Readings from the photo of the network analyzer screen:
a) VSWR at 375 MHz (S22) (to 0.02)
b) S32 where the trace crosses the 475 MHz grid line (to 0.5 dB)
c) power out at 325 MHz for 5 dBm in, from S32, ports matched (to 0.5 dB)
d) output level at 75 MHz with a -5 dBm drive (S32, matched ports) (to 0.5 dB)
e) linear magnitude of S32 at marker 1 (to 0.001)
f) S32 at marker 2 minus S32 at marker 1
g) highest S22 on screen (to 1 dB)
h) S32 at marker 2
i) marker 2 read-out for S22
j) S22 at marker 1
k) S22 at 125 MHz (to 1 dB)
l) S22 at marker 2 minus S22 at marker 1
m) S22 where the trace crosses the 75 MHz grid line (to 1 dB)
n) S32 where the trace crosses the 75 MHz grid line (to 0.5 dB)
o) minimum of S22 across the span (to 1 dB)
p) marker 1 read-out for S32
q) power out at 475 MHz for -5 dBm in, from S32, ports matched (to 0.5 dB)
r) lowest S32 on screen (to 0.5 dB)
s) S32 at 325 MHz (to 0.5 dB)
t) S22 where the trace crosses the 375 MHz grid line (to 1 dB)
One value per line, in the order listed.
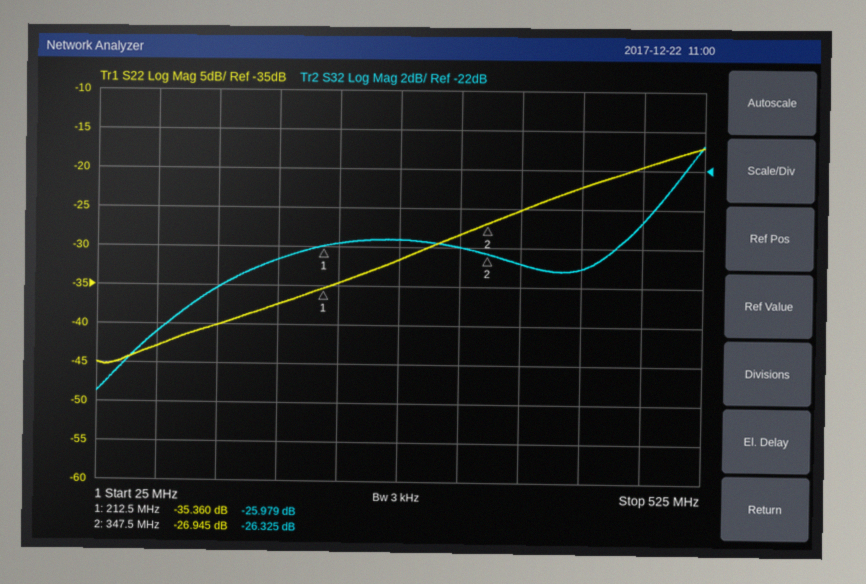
1.12
-24.5 dB
-21.0 dBm
-35.5 dBm
0.050
-0.346 dB
-17 dB
-26.325 dB
-26.945 dB
-35.360 dB
-40 dB
8.415 dB
-43 dB
-30.5 dB
-45 dB
-25.979 dB
-29.5 dBm
-33.5 dB
-26.0 dB
-25 dB
